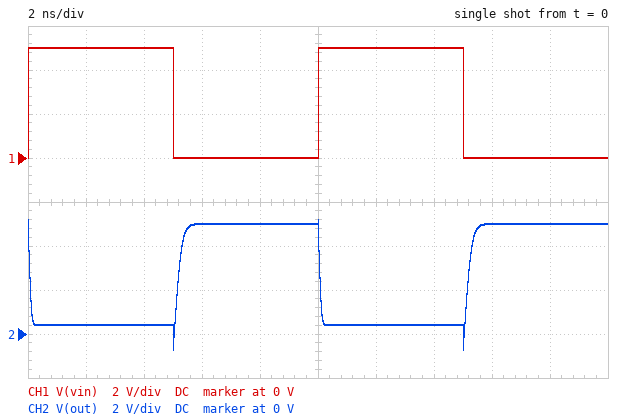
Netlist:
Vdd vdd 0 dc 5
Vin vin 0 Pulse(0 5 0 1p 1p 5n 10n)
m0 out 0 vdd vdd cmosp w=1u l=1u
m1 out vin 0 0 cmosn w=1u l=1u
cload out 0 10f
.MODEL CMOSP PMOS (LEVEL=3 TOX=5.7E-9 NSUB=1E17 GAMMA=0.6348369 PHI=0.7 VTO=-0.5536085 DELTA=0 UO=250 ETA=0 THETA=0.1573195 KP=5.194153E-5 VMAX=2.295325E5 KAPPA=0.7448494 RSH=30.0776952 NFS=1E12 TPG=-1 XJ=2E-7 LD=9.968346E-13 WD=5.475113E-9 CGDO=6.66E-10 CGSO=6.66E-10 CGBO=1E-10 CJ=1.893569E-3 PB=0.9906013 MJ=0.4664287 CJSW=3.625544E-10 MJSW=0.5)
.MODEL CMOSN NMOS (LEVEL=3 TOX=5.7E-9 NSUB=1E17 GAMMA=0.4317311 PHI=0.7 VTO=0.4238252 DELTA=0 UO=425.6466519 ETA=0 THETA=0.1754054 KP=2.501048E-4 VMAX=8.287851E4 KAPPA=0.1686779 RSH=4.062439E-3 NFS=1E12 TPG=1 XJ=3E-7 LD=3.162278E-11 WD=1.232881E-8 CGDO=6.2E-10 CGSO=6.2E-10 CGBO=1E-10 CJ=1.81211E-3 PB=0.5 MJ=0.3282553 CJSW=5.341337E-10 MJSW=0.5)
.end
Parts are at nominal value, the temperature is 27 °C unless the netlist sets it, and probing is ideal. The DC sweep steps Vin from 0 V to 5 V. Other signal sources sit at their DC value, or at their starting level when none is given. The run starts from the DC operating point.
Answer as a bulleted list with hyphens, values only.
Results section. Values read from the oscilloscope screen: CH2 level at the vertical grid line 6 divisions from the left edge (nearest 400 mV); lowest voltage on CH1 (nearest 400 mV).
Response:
- 400 mV
- 0 V
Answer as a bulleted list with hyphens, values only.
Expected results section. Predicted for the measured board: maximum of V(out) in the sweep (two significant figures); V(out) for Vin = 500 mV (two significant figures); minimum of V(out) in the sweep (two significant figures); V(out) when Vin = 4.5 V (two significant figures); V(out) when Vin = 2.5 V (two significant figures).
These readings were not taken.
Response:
- 5.0 V
- 5.0 V
- 400 mV
- 440 mV
- 1.2 V
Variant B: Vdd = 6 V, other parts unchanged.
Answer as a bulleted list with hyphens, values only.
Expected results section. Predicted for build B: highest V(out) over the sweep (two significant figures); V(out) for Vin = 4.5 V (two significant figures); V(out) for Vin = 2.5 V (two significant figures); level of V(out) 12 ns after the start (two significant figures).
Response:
- 6.0 V
- 640 mV
- 3.7 V
- 570 mV
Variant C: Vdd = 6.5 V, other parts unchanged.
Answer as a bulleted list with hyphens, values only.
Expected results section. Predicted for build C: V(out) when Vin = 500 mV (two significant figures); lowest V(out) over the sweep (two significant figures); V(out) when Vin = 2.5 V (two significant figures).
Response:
- 6.5 V
- 670 mV
- 4.4 V
